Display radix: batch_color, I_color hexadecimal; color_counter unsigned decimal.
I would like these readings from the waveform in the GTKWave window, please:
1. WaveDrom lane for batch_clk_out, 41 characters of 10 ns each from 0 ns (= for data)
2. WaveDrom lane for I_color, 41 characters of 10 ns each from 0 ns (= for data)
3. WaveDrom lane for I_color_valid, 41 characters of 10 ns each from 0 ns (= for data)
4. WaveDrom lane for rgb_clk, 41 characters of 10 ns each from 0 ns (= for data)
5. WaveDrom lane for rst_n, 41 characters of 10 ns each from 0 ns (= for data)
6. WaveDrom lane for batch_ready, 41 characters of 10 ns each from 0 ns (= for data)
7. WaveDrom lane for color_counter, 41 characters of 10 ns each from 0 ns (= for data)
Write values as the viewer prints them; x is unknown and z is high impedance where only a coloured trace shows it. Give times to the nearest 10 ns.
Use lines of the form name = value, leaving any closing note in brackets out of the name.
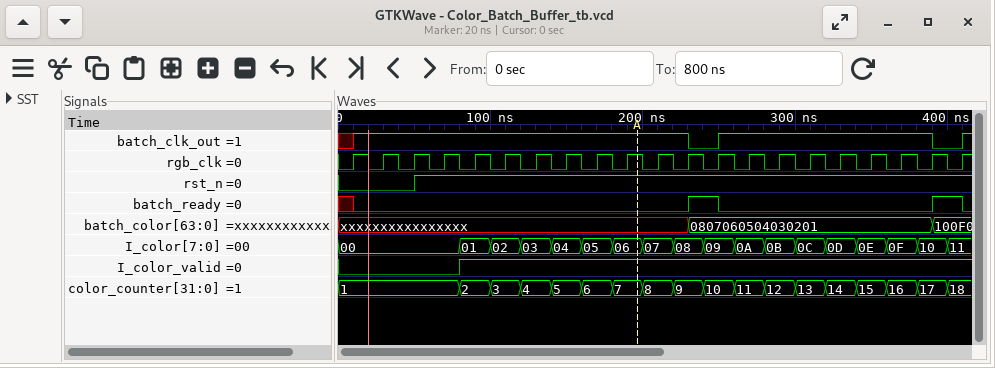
WaveDrom lane for batch_clk_out, 41 characters of 10 ns each from 0 ns = {name: 'batch_clk_out', wave: 'x1.....................0.1.............0.'}
WaveDrom lane for I_color, 41 characters of 10 ns each from 0 ns = {name: 'I_color', wave: '=.......=.=.=.=.=.=.=.=.=.=.=.=.=.=.=.=.=', data: '00 01 02 03 04 05 06 07 08 09 0A 0B 0C 0D 0E 0F 10 11'}
WaveDrom lane for I_color_valid, 41 characters of 10 ns each from 0 ns = {name: 'I_color_valid', wave: '0.......1................................'}
WaveDrom lane for rgb_clk, 41 characters of 10 ns each from 0 ns = {name: 'rgb_clk', wave: '01010101010101010101010101010101010101010'}
WaveDrom lane for rst_n, 41 characters of 10 ns each from 0 ns = {name: 'rst_n', wave: '0....1...................................'}
WaveDrom lane for batch_ready, 41 characters of 10 ns each from 0 ns = {name: 'batch_ready', wave: 'x0.....................1.0.............1.'}
WaveDrom lane for color_counter, 41 characters of 10 ns each from 0 ns = {name: 'color_counter', wave: '=.......=.=.=.=.=.=.=.=.=.=.=.=.=.=.=.=.=', data: '1 2 3 4 5 6 7 8 9 10 11 12 13 14 15 16 17 18'}
